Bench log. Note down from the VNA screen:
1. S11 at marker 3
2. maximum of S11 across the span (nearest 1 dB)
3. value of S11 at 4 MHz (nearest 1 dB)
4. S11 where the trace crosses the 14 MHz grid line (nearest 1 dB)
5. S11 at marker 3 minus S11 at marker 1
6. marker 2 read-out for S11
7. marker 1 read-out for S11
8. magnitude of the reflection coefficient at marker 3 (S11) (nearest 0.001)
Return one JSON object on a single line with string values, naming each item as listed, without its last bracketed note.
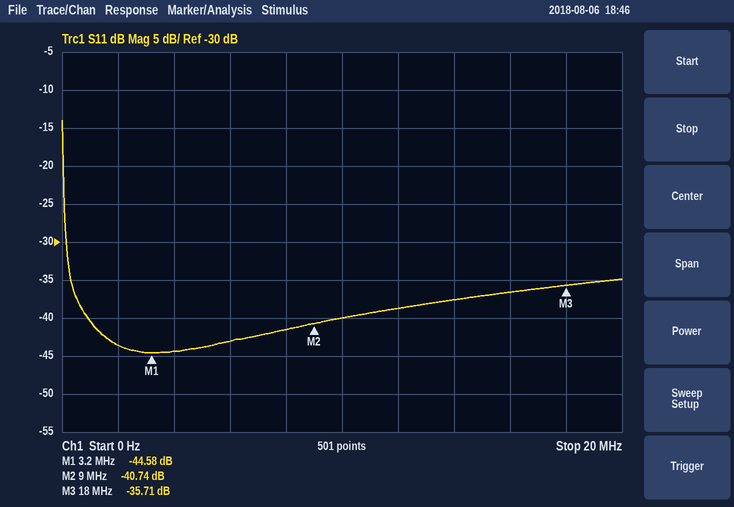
{"S11 at marker 3": "-35.71 dB", "maximum of S11 across the span": "-14 dB", "value of S11 at 4 MHz": "-44 dB", "S11 where the trace crosses the 14 MHz grid line": "-38 dB", "S11 at marker 3 minus S11 at marker 1": "8.87 dB", "marker 2 read-out for S11": "-40.74 dB", "marker 1 read-out for S11": "-44.58 dB", "magnitude of the reflection coefficient at marker 3 (S11)": "0.016"}
